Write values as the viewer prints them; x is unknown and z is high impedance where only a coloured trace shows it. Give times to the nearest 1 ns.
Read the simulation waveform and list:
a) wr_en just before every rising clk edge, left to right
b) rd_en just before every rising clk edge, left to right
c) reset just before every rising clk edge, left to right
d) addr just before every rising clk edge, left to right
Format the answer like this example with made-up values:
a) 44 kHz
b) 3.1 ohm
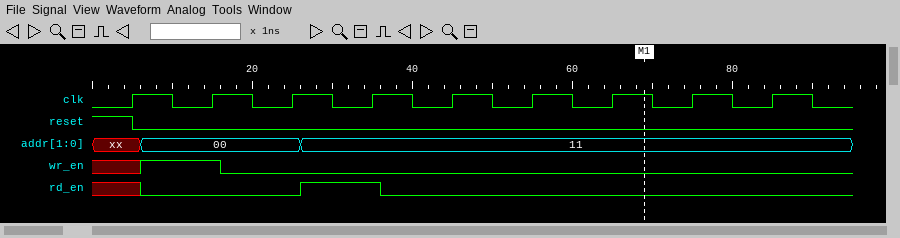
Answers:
a) x 1 0 0 0 0 0 0 0
b) x 0 0 1 0 0 0 0 0
c) 1 0 0 0 0 0 0 0 0
d) xx, 00, 00, 11, 11, 11, 11, 11, 11
